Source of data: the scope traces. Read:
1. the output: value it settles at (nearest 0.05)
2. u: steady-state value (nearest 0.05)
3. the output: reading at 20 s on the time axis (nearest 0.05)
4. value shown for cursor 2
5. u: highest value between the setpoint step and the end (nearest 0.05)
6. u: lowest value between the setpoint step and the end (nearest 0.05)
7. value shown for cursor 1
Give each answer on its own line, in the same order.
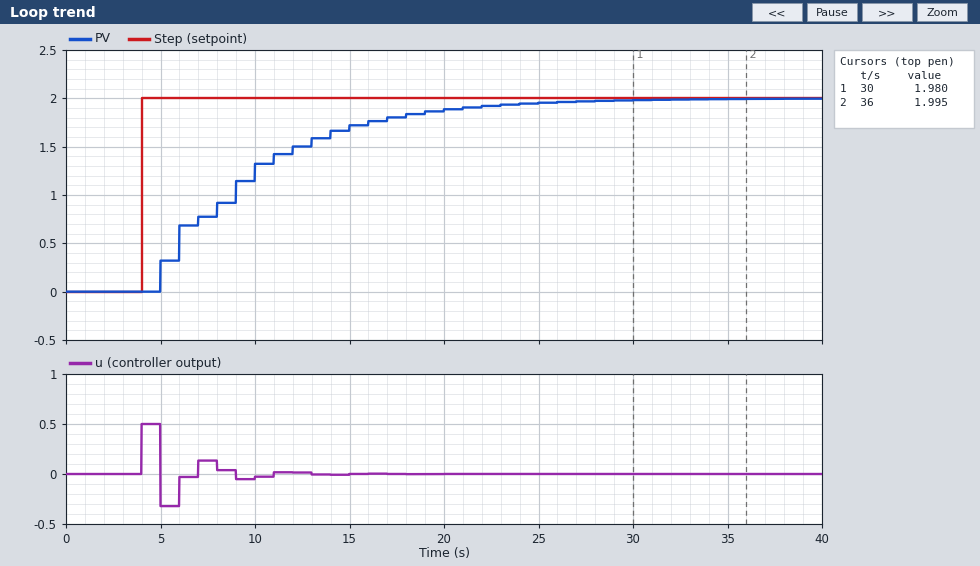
2.00
0.00
1.90
1.995
0.50
-0.30
1.980
